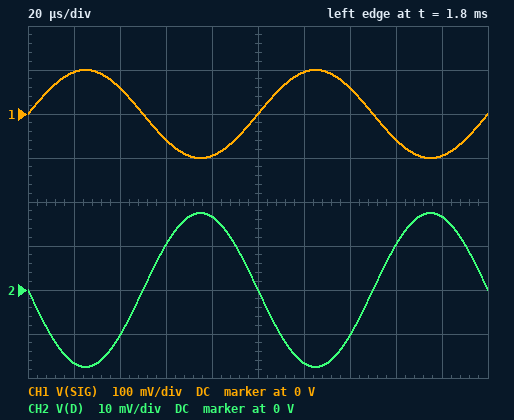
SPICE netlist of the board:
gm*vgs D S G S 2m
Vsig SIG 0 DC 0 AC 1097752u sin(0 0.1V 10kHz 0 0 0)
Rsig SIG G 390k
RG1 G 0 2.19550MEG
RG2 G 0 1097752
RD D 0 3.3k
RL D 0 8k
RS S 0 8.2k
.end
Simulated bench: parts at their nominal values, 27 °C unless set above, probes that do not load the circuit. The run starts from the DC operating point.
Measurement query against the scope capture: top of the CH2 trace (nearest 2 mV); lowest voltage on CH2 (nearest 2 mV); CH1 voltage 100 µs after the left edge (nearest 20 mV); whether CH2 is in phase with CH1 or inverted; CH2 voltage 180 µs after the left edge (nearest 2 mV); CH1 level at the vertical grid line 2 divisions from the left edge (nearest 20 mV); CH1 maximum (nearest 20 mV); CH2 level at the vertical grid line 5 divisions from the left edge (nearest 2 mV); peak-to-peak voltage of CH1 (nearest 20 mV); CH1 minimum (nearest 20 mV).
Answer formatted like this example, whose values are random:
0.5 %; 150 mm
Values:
18 mV; -18 mV; 0 V; inverted; 16 mV; 60 mV; 100 mV; 0 V; 200 mV; -100 mV
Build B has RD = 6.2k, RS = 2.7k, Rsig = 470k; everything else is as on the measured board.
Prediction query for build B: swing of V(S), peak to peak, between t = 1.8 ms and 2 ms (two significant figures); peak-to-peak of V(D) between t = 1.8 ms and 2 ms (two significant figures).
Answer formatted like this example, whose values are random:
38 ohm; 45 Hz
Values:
100 mV; 130 mV
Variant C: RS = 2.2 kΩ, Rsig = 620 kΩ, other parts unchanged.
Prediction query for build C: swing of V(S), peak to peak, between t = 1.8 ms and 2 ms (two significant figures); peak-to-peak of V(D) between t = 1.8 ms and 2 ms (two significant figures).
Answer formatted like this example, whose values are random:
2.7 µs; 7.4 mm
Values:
88 mV; 94 mV
